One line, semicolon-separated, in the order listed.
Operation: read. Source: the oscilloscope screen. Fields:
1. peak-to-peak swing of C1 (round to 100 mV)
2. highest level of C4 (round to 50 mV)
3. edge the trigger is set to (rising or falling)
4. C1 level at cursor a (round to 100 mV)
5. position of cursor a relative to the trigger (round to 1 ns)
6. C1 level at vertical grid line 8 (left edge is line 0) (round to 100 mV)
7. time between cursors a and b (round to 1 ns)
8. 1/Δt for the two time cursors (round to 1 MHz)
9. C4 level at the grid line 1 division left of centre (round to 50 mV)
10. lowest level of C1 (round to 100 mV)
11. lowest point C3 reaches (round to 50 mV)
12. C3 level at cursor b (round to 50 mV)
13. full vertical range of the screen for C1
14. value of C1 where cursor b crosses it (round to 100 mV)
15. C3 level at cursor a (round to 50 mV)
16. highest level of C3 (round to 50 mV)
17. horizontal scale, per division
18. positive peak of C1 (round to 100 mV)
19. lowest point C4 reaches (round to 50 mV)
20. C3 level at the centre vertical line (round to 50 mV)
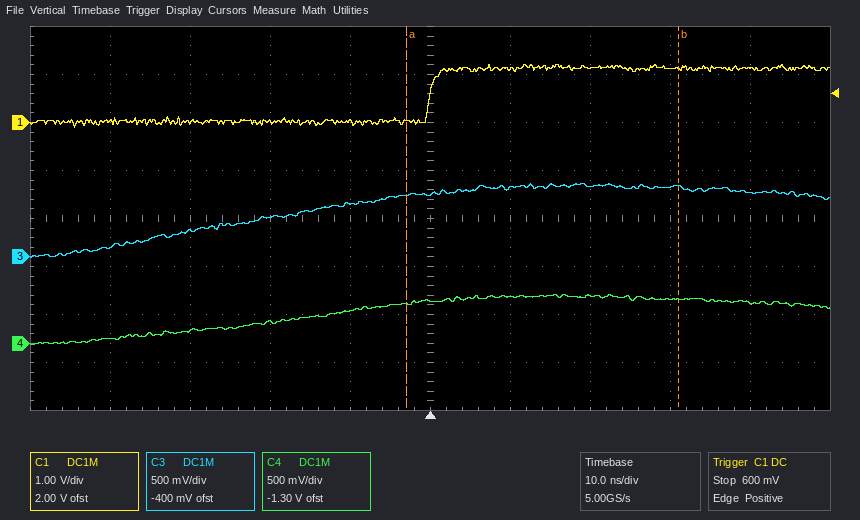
1.3 V; 500 mV; rising; 0.0 V; -3 ns; 1.1 V; 34 ns; 29 MHz; 350 mV; -100 mV; 0 mV; 750 mV; 8 V; 1.1 V; 650 mV; 750 mV; 10 ns; 1.2 V; 0 mV; 650 mV
